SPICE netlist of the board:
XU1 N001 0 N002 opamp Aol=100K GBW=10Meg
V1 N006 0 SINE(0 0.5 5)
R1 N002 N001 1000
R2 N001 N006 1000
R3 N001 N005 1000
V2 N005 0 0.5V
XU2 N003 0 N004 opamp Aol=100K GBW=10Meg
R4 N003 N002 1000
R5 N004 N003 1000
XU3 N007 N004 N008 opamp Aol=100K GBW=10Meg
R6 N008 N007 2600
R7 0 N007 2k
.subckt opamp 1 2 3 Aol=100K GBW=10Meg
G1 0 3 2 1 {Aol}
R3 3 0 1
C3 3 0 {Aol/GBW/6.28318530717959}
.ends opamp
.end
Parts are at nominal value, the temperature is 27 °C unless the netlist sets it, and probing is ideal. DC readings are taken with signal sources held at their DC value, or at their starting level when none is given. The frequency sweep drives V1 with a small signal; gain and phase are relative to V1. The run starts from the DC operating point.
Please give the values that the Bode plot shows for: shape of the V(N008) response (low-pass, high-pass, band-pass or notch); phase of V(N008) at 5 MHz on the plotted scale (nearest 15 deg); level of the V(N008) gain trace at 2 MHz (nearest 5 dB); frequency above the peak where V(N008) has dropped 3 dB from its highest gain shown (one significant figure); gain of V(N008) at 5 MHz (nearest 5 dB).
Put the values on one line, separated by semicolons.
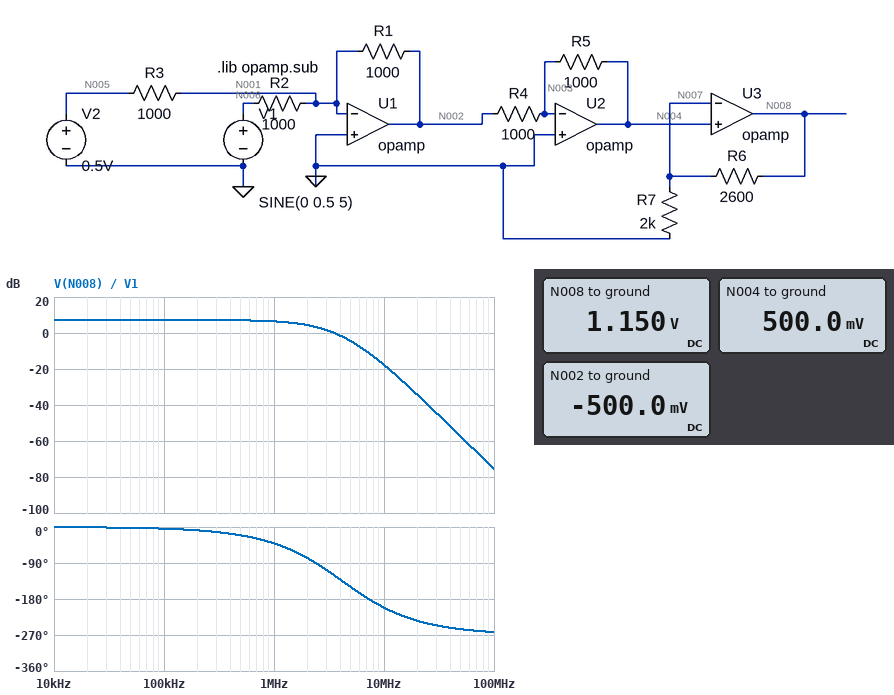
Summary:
low-pass; -150 deg; 5 dB; 2 MHz; -5 dB
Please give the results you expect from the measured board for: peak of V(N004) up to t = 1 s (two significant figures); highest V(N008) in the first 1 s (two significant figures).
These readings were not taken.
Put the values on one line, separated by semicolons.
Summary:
1.0 V; 2.3 V
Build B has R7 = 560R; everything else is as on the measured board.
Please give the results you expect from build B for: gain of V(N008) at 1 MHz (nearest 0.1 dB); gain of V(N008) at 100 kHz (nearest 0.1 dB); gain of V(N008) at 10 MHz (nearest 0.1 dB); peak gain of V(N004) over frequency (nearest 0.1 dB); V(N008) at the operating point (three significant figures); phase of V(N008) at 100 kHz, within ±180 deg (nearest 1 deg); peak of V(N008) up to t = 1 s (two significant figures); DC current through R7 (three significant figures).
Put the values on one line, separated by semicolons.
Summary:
13.3 dB; 15.0 dB; -17.1 dB; 0 dB; 2.82 V; -6 deg; 5.6 V; 893 µA
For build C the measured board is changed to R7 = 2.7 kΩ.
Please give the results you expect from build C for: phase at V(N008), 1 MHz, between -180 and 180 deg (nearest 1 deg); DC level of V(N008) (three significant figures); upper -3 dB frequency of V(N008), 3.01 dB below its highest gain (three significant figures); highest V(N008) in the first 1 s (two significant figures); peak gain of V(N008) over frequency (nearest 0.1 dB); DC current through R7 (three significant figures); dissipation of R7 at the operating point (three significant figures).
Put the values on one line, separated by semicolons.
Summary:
-39 deg; 981 mV; 2.17 MHz; 2.0 V; 5.9 dB; 185 µA; 92.6 µW
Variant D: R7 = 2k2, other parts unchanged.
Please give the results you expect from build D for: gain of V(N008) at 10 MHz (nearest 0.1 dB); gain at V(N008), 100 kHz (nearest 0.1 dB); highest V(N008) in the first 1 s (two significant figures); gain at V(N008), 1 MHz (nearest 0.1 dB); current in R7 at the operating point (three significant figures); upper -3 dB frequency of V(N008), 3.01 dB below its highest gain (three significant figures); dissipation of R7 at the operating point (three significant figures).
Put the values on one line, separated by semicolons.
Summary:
-17.8 dB; 6.8 dB; 2.2 V; 6.0 dB; 227 µA; 2.11 MHz; 114 µW
